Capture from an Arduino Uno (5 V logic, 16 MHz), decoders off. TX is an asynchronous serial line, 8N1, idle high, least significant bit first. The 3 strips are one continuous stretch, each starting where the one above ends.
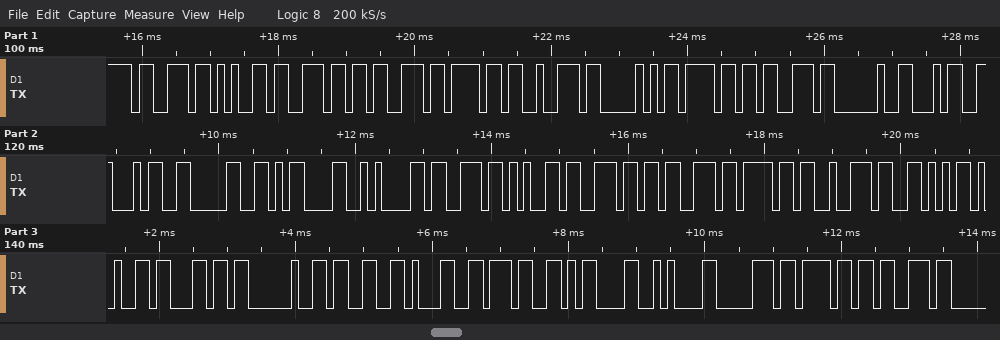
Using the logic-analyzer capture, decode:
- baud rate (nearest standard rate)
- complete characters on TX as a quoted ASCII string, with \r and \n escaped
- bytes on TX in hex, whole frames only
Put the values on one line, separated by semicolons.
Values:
9600 baud; "sensorPos 440\r\nsensorVel 317\r\npos"; 73 65 6E 73 6F 72 50 6F 73 20 34 34 30 0D 0A 73 65 6E 73 6F 72 56 65 6C 20 33 31 37 0D 0A 70 6F 73
